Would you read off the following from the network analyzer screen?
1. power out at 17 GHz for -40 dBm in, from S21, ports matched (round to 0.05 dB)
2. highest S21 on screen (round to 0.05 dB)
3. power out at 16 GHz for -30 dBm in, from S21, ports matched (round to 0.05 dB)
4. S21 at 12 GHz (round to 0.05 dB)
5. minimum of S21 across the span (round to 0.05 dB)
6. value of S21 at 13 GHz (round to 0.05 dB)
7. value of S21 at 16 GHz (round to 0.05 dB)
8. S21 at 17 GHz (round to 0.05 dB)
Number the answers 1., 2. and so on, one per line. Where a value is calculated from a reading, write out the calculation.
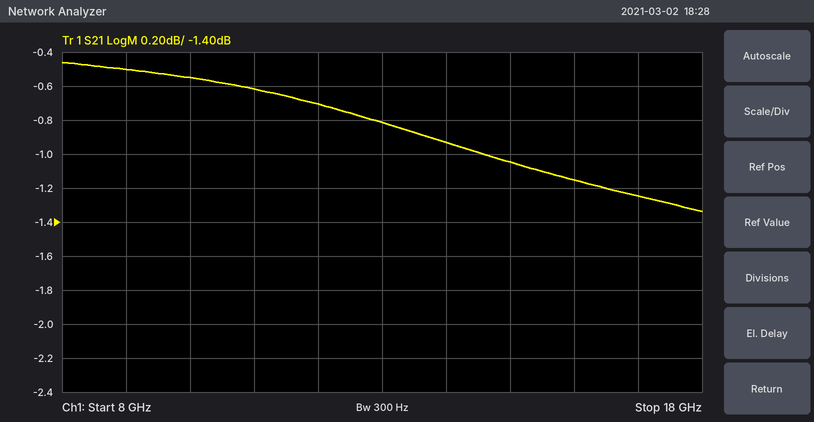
1. -40 dBm + (-1.25 dB) = -41.25 dBm
2. -0.45 dB
3. -30 dBm + (-1.15 dB) = -31.15 dBm
4. -0.70 dB
5. -1.35 dB
6. -0.80 dB
7. -1.15 dB
8. -1.25 dB
